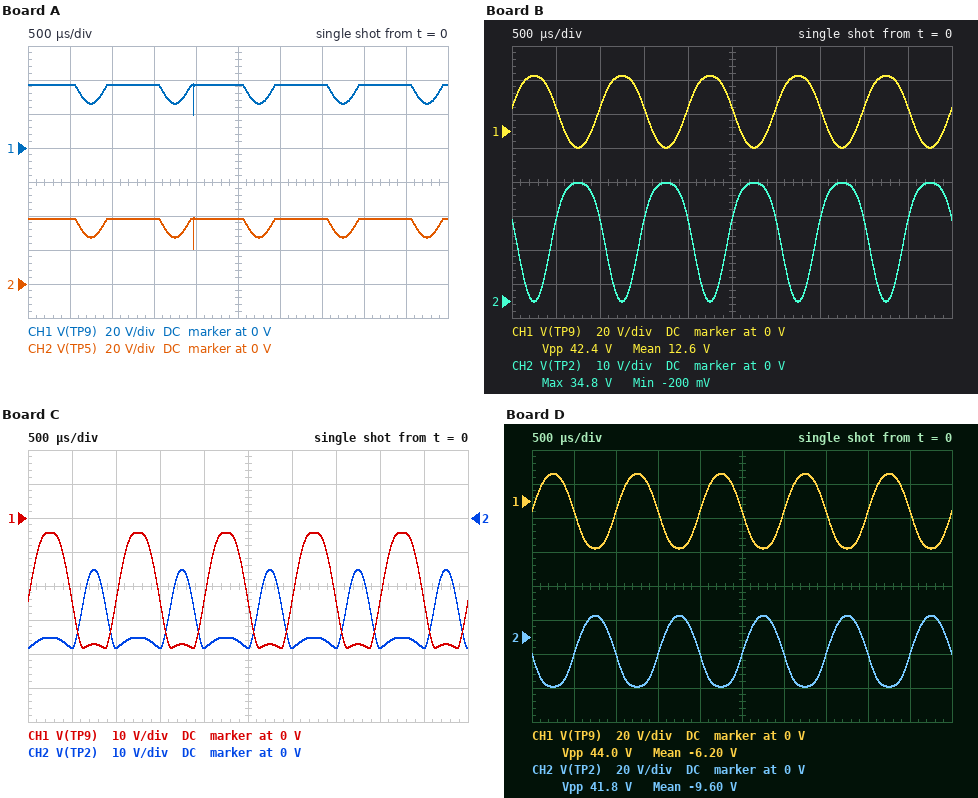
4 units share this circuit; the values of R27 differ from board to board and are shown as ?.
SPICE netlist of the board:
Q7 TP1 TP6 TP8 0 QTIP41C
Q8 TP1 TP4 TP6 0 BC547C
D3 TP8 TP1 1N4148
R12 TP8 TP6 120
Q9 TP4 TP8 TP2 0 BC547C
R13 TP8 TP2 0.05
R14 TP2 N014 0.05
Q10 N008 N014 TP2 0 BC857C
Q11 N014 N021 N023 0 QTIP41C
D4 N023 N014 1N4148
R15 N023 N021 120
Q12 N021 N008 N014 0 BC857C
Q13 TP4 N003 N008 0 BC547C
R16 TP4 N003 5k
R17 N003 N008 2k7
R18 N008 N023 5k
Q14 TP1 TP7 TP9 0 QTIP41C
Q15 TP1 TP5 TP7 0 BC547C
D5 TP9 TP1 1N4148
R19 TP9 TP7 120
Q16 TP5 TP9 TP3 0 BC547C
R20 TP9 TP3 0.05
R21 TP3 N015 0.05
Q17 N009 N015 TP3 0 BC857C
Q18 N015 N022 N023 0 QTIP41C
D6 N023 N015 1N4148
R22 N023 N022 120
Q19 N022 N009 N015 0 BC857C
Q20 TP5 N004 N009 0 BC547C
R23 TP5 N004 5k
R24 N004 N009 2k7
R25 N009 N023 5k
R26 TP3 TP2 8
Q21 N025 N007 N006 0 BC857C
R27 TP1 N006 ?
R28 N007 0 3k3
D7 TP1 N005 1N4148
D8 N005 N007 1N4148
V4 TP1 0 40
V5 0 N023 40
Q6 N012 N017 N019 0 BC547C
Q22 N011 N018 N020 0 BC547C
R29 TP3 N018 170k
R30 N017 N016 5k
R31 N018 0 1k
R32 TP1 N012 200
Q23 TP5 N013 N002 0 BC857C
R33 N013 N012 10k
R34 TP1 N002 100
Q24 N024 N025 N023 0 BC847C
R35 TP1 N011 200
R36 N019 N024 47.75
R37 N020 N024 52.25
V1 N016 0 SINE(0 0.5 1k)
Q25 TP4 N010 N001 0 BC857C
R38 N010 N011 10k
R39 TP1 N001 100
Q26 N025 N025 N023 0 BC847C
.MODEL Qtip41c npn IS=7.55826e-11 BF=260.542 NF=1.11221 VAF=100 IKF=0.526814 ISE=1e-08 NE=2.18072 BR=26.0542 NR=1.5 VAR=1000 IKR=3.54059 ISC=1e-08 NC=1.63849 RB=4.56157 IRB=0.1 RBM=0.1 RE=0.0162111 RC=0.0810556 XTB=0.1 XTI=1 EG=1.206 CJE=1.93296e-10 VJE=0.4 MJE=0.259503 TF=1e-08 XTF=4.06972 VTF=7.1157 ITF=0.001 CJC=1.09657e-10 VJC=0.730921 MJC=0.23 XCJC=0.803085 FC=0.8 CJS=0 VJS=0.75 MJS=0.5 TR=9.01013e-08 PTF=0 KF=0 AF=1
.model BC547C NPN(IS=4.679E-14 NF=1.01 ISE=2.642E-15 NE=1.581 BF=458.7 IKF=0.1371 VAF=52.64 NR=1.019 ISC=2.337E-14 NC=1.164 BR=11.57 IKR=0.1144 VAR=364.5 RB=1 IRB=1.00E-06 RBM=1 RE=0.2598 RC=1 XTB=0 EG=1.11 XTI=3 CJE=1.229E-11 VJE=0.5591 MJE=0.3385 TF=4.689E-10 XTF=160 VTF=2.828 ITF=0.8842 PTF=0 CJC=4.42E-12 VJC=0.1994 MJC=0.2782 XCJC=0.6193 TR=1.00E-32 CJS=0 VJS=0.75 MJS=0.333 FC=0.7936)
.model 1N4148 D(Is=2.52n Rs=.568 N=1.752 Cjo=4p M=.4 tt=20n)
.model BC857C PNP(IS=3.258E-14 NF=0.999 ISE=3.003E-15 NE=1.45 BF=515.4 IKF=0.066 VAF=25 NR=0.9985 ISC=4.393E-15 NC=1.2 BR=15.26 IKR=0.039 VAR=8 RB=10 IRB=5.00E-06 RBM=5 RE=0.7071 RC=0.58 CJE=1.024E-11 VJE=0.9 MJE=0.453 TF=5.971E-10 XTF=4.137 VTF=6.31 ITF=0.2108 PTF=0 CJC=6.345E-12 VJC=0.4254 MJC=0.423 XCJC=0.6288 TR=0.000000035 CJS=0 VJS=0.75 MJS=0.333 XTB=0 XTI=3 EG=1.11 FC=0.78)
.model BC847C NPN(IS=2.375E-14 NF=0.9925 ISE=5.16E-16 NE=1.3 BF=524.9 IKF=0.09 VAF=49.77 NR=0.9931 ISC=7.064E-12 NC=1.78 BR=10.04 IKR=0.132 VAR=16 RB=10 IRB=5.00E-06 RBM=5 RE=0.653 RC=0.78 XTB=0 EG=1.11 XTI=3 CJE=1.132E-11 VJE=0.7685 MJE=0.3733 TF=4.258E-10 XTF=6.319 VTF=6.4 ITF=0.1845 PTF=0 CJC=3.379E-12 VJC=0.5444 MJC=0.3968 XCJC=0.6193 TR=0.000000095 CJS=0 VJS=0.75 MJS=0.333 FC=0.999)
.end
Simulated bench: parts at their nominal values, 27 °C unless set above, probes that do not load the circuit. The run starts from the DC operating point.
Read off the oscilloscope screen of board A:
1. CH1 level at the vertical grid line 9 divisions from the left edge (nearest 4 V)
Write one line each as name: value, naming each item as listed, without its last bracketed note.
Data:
CH1 level at the vertical grid line 9 divisions from the left edge: 36 V
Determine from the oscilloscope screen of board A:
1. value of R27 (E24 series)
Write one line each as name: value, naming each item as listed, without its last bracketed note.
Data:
value of R27: 30 Ω
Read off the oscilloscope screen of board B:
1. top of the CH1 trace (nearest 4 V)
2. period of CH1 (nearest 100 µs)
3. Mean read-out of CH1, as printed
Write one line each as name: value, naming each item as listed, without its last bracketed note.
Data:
top of the CH1 trace: 32 V
period of CH1: 1.0 ms
Mean read-out of CH1, as printed: 12.6 V
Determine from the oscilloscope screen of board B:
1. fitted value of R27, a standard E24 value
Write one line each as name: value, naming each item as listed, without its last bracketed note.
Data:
fitted value of R27, a standard E24 value: 56 Ω
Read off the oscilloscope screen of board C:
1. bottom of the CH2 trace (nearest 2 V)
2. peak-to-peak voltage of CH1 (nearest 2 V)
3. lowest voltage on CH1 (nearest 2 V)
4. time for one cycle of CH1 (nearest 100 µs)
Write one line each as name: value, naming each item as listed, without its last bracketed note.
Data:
bottom of the CH2 trace: -38 V
peak-to-peak voltage of CH1: 34 V
lowest voltage on CH1: -38 V
time for one cycle of CH1: 1.0 ms
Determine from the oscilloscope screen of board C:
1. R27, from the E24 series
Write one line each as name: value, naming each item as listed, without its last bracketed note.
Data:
R27, from the E24 series: 180 Ω
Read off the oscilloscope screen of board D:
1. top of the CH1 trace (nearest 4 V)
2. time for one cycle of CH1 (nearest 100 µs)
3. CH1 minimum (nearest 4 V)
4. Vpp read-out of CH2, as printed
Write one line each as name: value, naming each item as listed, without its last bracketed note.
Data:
top of the CH1 trace: 16 V
time for one cycle of CH1: 1.0 ms
CH1 minimum: -28 V
Vpp read-out of CH2, as printed: 41.8 V
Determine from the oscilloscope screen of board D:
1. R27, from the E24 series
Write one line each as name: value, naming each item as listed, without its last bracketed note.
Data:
R27, from the E24 series: 91 Ω
